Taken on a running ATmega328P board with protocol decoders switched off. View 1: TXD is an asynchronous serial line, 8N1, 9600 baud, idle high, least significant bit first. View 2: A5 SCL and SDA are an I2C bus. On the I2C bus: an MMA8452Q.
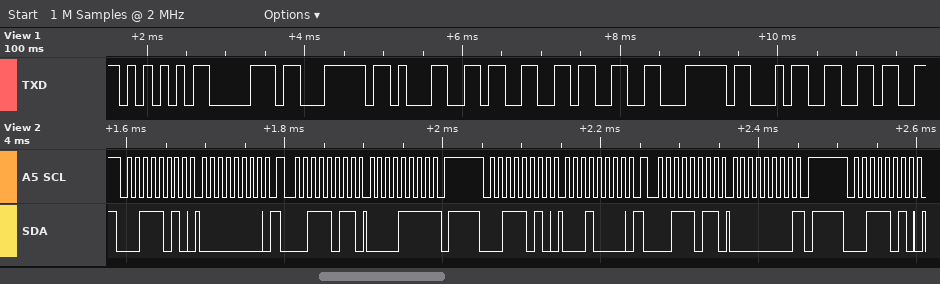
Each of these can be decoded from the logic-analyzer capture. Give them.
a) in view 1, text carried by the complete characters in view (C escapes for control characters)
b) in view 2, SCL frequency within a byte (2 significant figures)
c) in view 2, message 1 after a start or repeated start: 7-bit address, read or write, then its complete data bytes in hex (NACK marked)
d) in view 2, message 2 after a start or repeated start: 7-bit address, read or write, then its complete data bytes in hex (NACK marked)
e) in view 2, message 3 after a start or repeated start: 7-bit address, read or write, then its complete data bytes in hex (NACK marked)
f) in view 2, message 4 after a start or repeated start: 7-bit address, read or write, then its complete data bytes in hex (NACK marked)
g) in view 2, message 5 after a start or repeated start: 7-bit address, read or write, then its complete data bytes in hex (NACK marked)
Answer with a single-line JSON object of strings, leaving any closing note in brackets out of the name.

{"in view 1, text carried by the complete characters in view": "\"Up|133|46\"", "in view 2, SCL frequency within a byte": "100 kHz", "in view 2, message 1 after a start or repeated start: 7-bit address, read or write, then its complete data bytes in hex": "0x1D write: 00", "in view 2, message 2 after a start or repeated start: 7-bit address, read or write, then its complete data bytes in hex": "0x1D read: 0F NACK", "in view 2, message 3 after a start or repeated start: 7-bit address, read or write, then its complete data bytes in hex": "0x1D write: 10", "in view 2, message 4 after a start or repeated start: 7-bit address, read or write, then its complete data bytes in hex": "0x1D read: 00 NACK", "in view 2, message 5 after a start or repeated start: 7-bit address, read or write, then its complete data bytes in hex": "0x1D write"}
